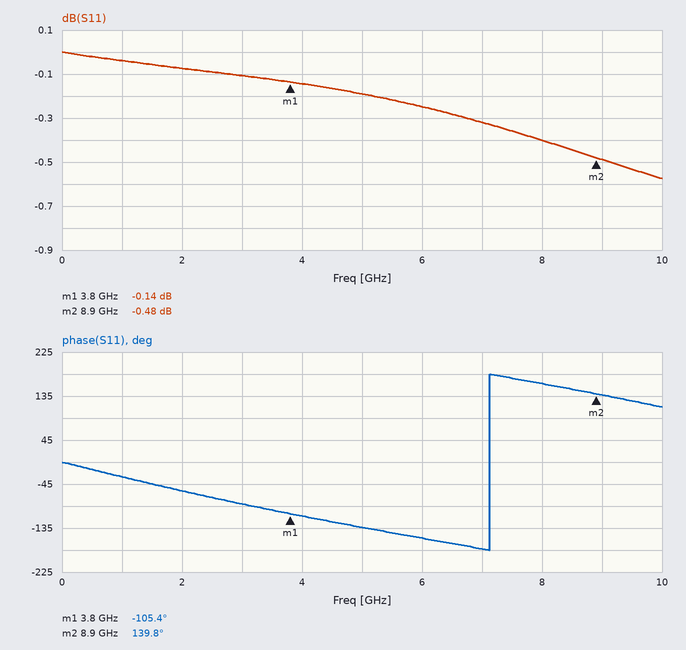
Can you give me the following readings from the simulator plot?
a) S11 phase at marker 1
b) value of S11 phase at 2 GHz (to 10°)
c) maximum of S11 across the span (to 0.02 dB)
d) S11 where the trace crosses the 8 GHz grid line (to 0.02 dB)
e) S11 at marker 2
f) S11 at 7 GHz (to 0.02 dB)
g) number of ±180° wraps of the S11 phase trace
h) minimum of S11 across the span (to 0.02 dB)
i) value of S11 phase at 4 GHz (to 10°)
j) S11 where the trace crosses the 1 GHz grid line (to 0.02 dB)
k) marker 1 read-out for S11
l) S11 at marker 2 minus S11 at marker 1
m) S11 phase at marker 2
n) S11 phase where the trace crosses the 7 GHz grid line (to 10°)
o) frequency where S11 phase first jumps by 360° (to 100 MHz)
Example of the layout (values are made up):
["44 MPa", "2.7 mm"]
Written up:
["-105.4°", "-60°", "0.00 dB", "-0.40 dB", "-0.48 dB", "-0.32 dB", "1", "-0.58 dB", "-110°", "-0.04 dB", "-0.14 dB", "-0.34 dB", "139.8°", "-180°", "7.1 GHz"]
